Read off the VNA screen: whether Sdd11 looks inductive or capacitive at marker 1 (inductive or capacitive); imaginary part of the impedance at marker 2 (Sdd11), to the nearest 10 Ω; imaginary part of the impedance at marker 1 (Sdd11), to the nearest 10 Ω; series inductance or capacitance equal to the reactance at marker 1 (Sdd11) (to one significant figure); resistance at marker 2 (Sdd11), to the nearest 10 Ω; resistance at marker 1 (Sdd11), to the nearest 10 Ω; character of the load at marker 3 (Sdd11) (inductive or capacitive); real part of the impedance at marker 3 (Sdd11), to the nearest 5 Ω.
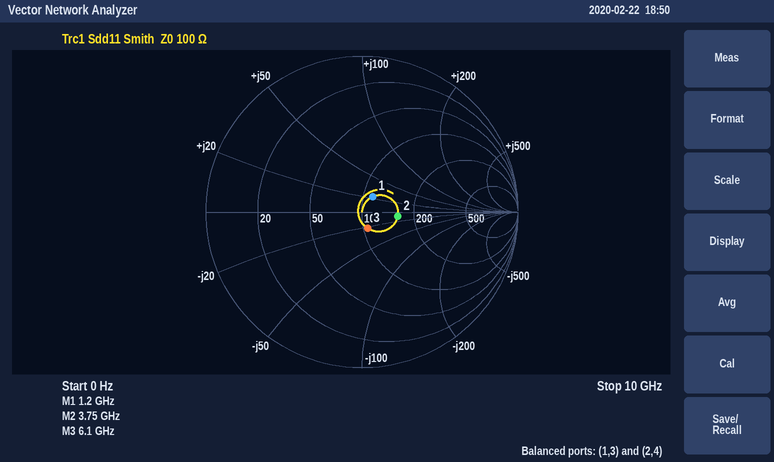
inductive
-10 Ω
+20 Ω
3 nH
160 Ω
110 Ω
capacitive
105 Ω
